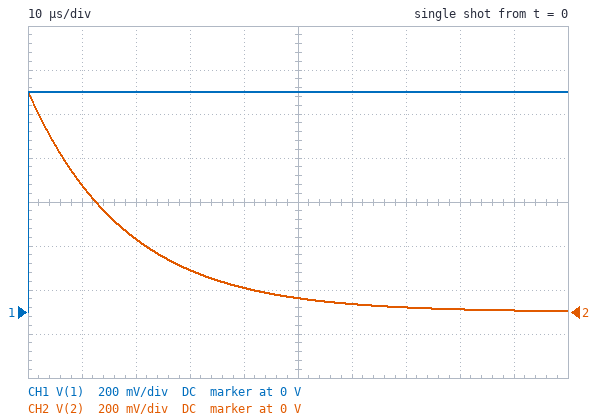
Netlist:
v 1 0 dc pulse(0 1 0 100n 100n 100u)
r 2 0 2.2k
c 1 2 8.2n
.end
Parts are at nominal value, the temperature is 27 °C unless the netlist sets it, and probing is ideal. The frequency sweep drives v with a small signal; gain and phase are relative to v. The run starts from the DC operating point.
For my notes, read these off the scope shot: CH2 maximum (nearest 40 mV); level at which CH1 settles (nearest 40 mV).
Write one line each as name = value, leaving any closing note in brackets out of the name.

CH2 maximum = 1.00 V
level at which CH1 settles = 1.00 V
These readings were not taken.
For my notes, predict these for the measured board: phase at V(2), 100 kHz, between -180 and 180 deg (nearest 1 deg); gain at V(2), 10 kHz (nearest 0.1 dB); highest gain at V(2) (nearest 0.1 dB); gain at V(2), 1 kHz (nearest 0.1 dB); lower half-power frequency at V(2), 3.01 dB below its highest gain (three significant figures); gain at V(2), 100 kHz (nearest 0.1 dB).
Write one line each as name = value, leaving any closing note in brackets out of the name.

phase at V(2), 100 kHz, between -180 and 180 deg = 5 deg
gain at V(2), 10 kHz = -2.5 dB
highest gain at V(2) = 0 dB
gain at V(2), 1 kHz = -19.0 dB
lower half-power frequency at V(2), 3.01 dB below its highest gain = 8.82 kHz
gain at V(2), 100 kHz = 0 dB
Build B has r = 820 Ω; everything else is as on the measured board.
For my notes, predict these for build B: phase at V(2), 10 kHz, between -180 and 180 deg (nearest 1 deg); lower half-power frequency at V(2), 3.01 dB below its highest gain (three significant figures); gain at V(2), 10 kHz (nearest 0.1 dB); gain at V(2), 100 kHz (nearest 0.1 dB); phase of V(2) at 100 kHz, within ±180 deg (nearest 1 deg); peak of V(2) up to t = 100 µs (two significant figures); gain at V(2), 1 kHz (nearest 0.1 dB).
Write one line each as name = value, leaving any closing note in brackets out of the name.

phase at V(2), 10 kHz, between -180 and 180 deg = 67 deg
lower half-power frequency at V(2), 3.01 dB below its highest gain = 23.7 kHz
gain at V(2), 10 kHz = -8.2 dB
gain at V(2), 100 kHz = -0.2 dB
phase of V(2) at 100 kHz, within ±180 deg = 13 deg
peak of V(2) up to t = 100 µs = 990 mV
gain at V(2), 1 kHz = -27.5 dB
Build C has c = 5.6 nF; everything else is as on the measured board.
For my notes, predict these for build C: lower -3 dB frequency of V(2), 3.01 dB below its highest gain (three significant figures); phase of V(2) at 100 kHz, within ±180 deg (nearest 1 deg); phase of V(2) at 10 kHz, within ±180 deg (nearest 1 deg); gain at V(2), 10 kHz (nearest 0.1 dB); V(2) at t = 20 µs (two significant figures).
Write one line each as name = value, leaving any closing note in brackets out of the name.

lower -3 dB frequency of V(2), 3.01 dB below its highest gain = 12.9 kHz
phase of V(2) at 100 kHz, within ±180 deg = 7 deg
phase of V(2) at 10 kHz, within ±180 deg = 52 deg
gain at V(2), 10 kHz = -4.3 dB
V(2) at t = 20 µs = 200 mV
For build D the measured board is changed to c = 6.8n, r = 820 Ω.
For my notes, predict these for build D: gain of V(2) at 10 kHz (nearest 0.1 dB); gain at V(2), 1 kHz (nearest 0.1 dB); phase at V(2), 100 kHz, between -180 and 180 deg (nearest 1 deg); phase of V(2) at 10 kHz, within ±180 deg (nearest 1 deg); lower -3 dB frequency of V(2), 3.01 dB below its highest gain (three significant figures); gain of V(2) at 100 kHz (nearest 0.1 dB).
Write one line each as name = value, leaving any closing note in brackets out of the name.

gain of V(2) at 10 kHz = -9.6 dB
gain at V(2), 1 kHz = -29.1 dB
phase at V(2), 100 kHz, between -180 and 180 deg = 16 deg
phase of V(2) at 10 kHz, within ±180 deg = 71 deg
lower -3 dB frequency of V(2), 3.01 dB below its highest gain = 28.5 kHz
gain of V(2) at 100 kHz = -0.3 dB
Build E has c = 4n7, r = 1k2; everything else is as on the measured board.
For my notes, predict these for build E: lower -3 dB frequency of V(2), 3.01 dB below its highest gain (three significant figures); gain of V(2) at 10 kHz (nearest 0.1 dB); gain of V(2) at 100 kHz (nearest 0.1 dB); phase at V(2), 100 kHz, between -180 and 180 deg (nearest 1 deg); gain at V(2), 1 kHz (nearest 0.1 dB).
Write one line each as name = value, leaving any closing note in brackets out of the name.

lower -3 dB frequency of V(2), 3.01 dB below its highest gain = 28.2 kHz
gain of V(2) at 10 kHz = -9.5 dB
gain of V(2) at 100 kHz = -0.3 dB
phase at V(2), 100 kHz, between -180 and 180 deg = 16 deg
gain at V(2), 1 kHz = -29.0 dB
